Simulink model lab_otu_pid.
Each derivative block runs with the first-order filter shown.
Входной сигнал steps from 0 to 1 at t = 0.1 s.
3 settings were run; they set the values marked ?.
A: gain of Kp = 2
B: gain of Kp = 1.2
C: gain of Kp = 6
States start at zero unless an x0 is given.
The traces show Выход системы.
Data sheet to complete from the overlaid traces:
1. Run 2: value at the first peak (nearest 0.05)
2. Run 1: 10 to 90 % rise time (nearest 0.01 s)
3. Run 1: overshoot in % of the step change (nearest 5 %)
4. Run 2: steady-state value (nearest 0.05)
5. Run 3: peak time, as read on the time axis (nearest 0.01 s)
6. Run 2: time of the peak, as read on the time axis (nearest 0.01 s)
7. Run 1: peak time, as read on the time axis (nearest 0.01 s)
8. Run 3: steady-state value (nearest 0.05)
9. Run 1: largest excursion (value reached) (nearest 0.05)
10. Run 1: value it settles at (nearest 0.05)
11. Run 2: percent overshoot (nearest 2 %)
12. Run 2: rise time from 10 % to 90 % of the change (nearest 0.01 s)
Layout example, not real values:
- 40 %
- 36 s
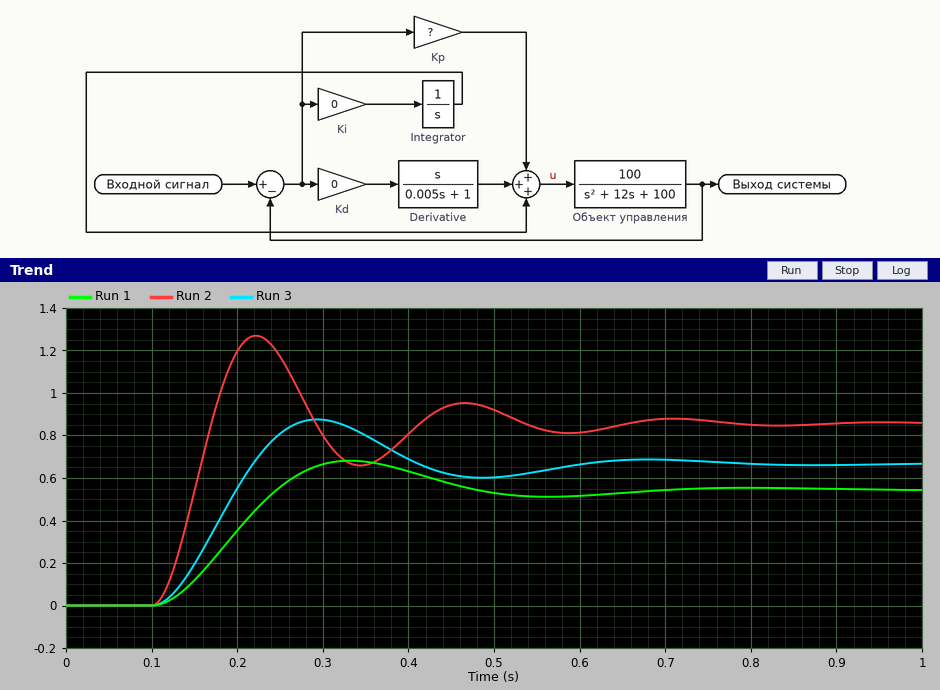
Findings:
- 1.25
- 0.10 s
- 25 %
- 0.85
- 0.29 s
- 0.22 s
- 0.33 s
- 0.65
- 0.70
- 0.55
- 48 %
- 0.05 s
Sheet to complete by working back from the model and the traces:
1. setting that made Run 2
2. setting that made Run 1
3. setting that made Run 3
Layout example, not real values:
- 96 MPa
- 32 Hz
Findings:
- C
- B
- A
